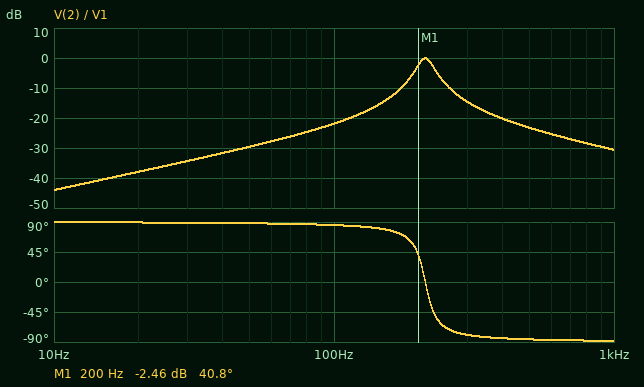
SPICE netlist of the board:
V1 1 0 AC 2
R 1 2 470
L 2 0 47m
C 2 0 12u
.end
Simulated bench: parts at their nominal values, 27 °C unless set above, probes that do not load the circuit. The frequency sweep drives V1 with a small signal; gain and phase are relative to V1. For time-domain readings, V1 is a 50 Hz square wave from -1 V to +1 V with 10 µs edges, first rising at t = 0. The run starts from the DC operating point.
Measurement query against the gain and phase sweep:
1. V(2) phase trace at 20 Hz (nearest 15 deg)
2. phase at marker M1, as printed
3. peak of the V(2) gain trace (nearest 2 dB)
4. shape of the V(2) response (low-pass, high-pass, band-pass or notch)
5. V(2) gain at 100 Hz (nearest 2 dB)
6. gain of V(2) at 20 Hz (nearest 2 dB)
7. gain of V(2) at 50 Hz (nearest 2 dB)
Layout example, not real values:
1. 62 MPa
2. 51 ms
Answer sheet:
1. 90 deg
2. 40.8 deg
3. 0 dB
4. band-pass
5. -22 dB
6. -38 dB
7. -30 dB
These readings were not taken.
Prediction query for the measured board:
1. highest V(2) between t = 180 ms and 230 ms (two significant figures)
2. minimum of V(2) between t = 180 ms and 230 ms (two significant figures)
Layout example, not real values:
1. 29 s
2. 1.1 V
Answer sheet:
1. 180 mV
2. -180 mV
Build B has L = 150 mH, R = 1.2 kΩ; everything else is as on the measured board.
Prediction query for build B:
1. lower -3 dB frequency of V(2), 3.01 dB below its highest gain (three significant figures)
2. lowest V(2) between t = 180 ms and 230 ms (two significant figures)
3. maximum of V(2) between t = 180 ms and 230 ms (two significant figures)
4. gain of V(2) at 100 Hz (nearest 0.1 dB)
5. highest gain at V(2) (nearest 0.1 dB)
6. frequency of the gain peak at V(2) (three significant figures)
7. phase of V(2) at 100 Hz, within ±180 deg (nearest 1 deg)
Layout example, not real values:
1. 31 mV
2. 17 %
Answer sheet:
1. 113 Hz
2. -120 mV
3. 120 mV
4. -11.6 dB
5. 0 dB
6. 119 Hz
7. 75 deg
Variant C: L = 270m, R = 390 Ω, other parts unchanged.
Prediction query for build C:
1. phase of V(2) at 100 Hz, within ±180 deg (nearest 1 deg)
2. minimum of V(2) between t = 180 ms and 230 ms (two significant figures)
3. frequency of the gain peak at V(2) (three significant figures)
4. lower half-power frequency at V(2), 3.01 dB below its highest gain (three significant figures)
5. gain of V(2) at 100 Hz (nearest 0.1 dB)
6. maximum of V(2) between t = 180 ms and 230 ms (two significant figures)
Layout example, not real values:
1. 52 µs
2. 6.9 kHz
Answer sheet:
1. -33 deg
2. -490 mV
3. 88.4 Hz
4. 73.0 Hz
5. -1.5 dB
6. 490 mV
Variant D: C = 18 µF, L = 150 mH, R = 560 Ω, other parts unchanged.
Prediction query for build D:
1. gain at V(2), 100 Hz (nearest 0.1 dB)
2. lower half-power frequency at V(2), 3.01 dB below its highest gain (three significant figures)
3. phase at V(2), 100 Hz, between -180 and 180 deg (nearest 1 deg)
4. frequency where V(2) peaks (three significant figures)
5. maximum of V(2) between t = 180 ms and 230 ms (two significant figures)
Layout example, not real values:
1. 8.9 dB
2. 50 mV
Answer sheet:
1. -0.6 dB
2. 89.3 Hz
3. -21 deg
4. 96.9 Hz
5. 180 mV
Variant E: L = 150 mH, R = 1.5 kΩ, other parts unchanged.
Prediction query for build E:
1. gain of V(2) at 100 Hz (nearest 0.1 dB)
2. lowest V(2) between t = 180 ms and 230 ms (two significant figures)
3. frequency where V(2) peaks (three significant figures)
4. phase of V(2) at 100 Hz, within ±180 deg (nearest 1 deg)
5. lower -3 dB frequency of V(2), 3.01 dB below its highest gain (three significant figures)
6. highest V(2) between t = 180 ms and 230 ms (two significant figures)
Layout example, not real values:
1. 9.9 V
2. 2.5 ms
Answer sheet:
1. -13.5 dB
2. -94 mV
3. 119 Hz
4. 78 deg
5. 114 Hz
6. 94 mV
